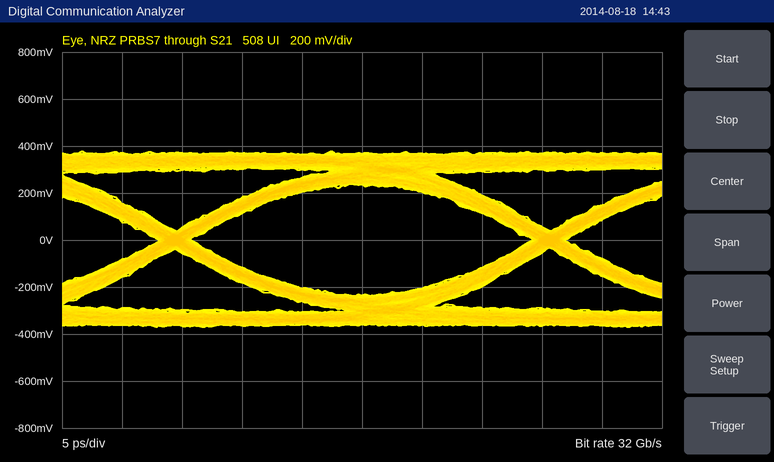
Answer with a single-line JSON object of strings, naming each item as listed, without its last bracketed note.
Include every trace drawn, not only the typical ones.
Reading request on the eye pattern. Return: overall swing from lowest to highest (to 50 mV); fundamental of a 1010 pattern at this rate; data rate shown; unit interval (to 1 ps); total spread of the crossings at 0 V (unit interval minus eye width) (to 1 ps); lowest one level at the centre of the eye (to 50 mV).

{"overall swing from lowest to highest": "750 mV", "fundamental of a 1010 pattern at this rate": "16 GHz", "data rate shown": "32 Gb/s", "unit interval": "31 ps", "total spread of the crossings at 0 V (unit interval minus eye width)": "3 ps", "lowest one level at the centre of the eye": "250 mV"}
